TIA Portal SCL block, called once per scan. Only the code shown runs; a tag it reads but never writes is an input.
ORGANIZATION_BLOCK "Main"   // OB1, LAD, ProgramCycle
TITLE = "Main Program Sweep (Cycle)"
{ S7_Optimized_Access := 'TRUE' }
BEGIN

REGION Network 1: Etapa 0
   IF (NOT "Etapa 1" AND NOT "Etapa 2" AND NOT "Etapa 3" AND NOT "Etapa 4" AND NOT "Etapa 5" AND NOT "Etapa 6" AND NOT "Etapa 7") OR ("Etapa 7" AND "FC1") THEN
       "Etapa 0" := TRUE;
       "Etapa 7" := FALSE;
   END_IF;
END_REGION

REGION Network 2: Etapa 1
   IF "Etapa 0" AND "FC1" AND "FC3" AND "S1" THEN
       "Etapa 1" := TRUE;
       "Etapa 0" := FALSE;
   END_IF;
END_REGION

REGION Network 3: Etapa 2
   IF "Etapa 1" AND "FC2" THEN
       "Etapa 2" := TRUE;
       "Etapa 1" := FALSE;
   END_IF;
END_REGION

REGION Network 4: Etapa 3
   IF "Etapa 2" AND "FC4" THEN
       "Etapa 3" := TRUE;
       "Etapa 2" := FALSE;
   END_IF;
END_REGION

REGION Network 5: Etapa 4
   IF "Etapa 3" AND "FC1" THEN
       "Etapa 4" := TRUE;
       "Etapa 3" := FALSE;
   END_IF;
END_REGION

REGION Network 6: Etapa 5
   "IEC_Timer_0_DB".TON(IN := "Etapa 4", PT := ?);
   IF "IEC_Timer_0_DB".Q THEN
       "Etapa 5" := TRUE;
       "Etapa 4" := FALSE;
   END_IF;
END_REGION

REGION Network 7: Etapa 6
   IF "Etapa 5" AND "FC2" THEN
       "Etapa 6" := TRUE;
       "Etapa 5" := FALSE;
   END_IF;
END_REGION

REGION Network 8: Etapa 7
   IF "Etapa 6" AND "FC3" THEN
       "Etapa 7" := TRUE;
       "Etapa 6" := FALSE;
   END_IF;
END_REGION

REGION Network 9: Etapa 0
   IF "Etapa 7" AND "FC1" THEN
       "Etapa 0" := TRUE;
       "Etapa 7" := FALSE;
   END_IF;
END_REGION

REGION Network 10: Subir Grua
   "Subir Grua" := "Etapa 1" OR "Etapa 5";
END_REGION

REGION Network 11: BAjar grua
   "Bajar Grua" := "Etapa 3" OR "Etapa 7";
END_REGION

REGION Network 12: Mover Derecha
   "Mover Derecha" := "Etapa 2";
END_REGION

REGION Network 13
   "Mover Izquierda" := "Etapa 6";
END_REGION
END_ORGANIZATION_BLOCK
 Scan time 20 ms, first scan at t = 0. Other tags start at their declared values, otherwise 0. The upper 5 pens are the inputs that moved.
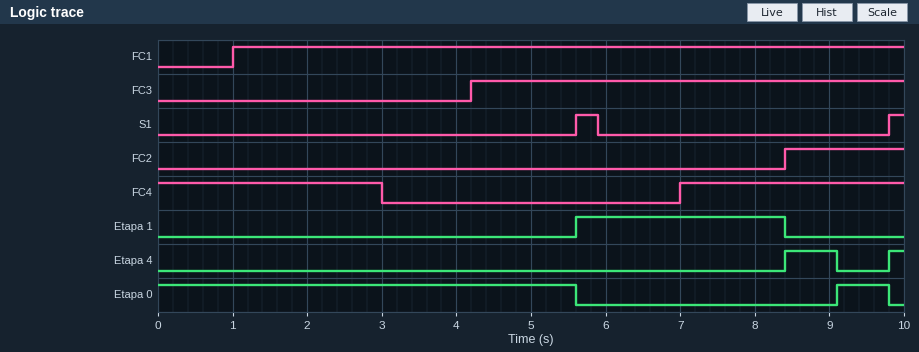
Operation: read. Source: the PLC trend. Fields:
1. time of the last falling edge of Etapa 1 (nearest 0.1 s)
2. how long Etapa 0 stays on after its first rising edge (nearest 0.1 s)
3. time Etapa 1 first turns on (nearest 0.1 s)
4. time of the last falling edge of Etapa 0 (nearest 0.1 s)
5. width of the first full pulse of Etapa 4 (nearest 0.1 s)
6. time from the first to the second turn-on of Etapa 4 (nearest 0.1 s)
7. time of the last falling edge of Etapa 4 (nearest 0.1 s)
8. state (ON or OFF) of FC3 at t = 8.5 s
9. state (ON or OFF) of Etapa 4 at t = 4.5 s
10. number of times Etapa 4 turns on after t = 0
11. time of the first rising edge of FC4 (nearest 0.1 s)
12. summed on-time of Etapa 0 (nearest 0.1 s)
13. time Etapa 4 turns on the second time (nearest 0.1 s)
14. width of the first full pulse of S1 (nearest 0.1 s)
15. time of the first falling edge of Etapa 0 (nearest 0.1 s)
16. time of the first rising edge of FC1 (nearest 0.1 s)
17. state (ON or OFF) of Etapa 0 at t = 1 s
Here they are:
8.4 s
0.7 s
5.6 s
9.8 s
0.7 s
1.4 s
9.1 s
ON
OFF
2
7.0 s
6.3 s
9.8 s
0.3 s
5.6 s
1.0 s
ON
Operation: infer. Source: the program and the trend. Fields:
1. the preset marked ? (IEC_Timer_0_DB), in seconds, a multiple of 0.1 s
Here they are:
0.7 s
